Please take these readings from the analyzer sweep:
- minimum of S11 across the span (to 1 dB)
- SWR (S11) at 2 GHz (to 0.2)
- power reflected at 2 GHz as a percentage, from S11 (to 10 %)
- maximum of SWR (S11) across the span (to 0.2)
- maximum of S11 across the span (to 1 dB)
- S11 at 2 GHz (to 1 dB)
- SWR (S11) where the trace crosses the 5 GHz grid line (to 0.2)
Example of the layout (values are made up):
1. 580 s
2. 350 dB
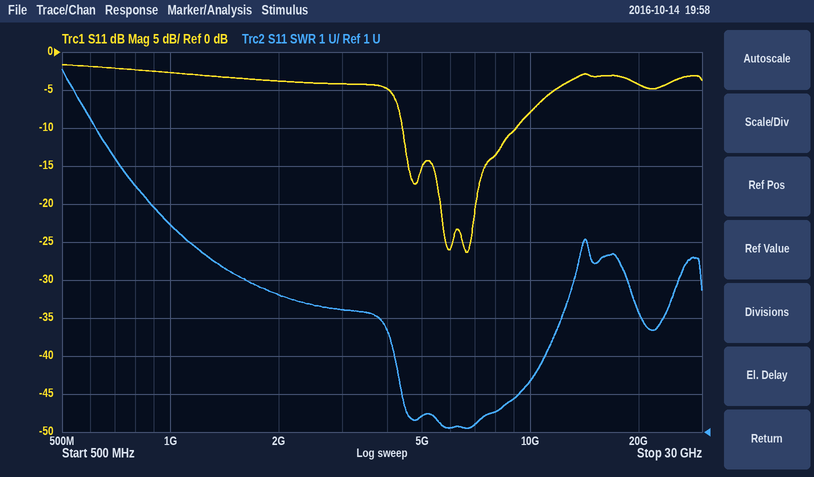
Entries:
1. -26 dB
2. 4.6
3. 40 %
4. 10.6
5. -2 dB
6. -4 dB
7. 1.4
